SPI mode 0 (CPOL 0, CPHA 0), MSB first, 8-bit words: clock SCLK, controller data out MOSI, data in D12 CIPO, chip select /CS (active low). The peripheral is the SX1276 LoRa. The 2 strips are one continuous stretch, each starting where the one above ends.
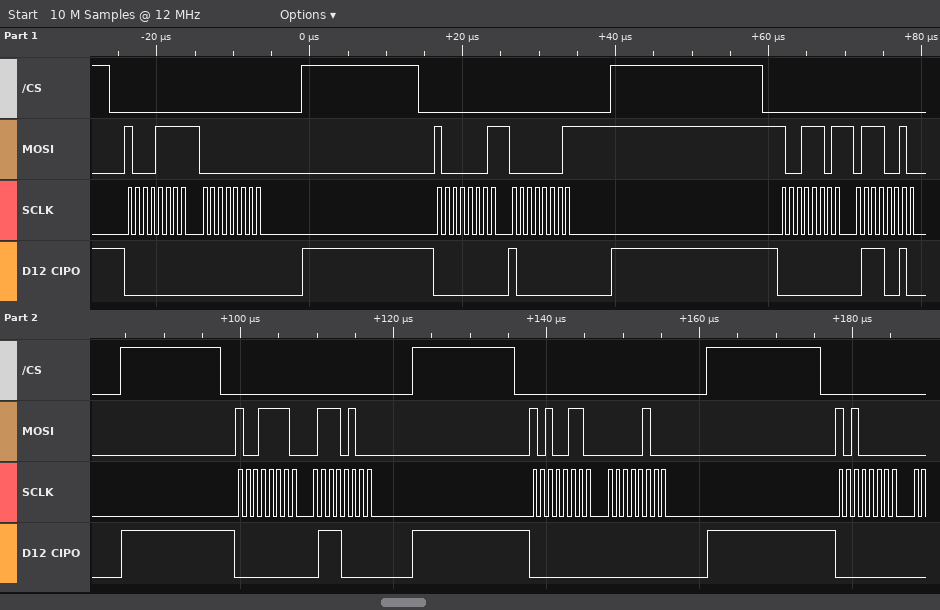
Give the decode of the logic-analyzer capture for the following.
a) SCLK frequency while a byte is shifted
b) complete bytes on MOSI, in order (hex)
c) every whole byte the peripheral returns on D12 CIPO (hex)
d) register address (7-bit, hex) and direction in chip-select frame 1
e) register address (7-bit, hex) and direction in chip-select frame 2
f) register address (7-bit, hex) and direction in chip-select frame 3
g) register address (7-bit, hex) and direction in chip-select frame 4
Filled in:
1 MHz
0x8F 0x00 0x81 0x01 0x9D 0x72 0x9E 0x74 0xA6 0x04 0xA0
0x00 0x00 0x00 0x80 0x00 0x72 0x00 0x70 0x00 0x00 0x00
0x0F write
0x01 write
0x1D write
0x1E write
